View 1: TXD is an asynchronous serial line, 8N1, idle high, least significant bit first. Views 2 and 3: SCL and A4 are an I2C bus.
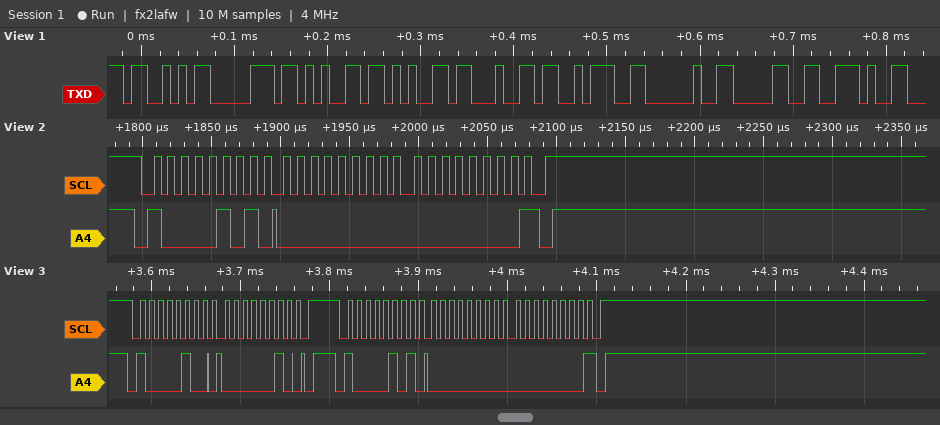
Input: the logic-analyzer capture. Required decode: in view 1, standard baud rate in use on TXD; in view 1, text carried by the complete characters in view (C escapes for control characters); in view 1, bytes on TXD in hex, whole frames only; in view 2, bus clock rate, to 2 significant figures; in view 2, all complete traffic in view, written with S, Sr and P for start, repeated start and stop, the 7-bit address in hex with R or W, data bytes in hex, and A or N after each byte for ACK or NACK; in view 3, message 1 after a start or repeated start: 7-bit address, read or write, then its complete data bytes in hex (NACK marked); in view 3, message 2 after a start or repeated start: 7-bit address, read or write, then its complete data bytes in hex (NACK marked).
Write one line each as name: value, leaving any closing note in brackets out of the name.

in view 1, standard baud rate in use on TXD: 115200 baud
in view 1, text carried by the complete characters in view: "Speed: 0."
in view 1, bytes on TXD in hex, whole frames only: 0x53 0x70 0x65 0x65 0x64 0x3A 0x20 0x30 0x2E
in view 2, bus clock rate, to 2 significant figures: 100 kHz
in view 2, all complete traffic in view, written with S, Sr and P for start, repeated start and stop, the 7-bit address in hex with R or W, data bytes in hex, and A or N after each byte for ACK or NACK: S 42R A 00 A 00 N P
in view 3, message 1 after a start or repeated start: 7-bit address, read or write, then its complete data bytes in hex: 0x42 write: 02
in view 3, message 2 after a start or repeated start: 7-bit address, read or write, then its complete data bytes in hex: 0x42 read: 00 00 NACK
